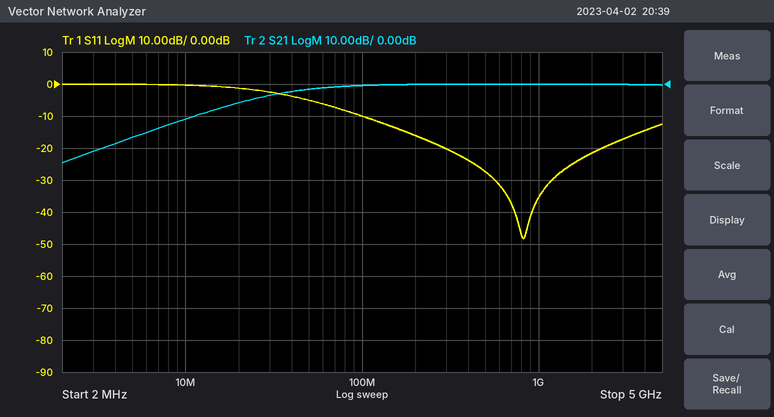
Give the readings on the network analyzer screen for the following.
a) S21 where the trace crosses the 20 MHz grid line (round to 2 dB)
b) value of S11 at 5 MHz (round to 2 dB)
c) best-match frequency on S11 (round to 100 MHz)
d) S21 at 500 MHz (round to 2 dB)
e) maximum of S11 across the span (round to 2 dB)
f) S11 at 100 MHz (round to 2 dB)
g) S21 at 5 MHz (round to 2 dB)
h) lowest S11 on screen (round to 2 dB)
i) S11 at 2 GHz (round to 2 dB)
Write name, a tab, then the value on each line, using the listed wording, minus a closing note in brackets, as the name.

S21 where the trace crosses the 20 MHz grid line	-6 dB
value of S11 at 5 MHz	0 dB
best-match frequency on S11	800 MHz
S21 at 500 MHz	0 dB
maximum of S11 across the span	0 dB
S11 at 100 MHz	-10 dB
S21 at 5 MHz	-16 dB
lowest S11 on screen	-48 dB
S11 at 2 GHz	-22 dB
